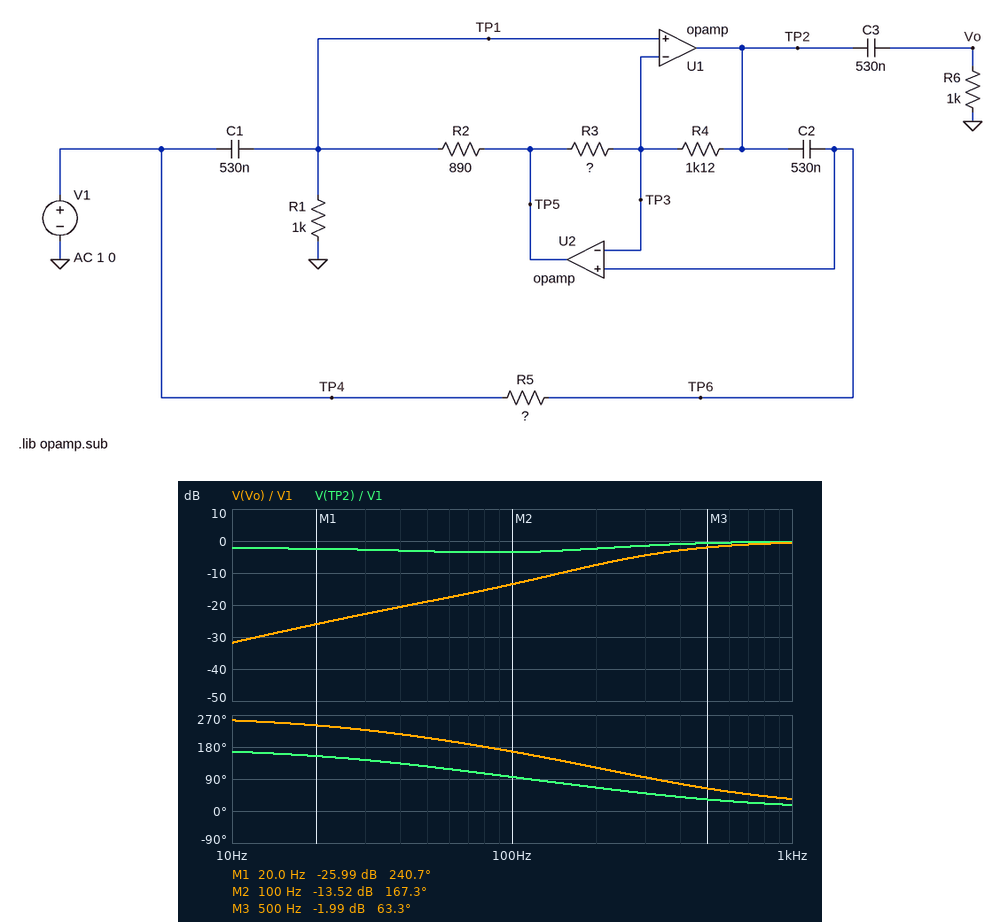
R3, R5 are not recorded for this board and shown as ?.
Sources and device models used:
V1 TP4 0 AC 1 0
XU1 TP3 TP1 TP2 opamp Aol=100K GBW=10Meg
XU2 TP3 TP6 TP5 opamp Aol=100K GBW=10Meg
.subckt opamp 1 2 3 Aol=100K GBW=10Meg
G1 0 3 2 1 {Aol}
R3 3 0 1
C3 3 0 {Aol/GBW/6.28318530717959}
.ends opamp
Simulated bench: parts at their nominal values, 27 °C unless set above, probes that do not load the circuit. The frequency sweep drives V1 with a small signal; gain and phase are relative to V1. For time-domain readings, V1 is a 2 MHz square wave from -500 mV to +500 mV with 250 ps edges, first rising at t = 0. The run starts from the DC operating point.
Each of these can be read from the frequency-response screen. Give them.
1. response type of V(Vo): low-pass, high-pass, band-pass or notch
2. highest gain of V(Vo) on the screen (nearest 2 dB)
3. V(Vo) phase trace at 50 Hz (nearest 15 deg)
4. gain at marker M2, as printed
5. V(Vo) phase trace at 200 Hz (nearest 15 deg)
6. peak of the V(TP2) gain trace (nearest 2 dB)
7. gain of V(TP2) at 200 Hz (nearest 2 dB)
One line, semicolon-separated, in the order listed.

high-pass; 0 dB; 210 deg; -13.52 dB; 120 deg; 0 dB; -2 dB
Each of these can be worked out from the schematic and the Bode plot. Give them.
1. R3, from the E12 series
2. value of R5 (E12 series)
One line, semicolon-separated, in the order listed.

560 Ω; 3.9 kΩ
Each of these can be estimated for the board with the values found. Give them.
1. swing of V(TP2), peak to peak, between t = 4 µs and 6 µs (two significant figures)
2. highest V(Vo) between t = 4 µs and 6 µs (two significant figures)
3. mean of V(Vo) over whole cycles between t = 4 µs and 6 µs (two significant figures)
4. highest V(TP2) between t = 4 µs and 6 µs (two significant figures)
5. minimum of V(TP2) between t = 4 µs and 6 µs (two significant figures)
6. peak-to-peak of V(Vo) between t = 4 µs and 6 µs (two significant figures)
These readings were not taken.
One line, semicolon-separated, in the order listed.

1.5 V; 1.2 V; 490 mV; 1.6 V; 140 mV; 1.5 V
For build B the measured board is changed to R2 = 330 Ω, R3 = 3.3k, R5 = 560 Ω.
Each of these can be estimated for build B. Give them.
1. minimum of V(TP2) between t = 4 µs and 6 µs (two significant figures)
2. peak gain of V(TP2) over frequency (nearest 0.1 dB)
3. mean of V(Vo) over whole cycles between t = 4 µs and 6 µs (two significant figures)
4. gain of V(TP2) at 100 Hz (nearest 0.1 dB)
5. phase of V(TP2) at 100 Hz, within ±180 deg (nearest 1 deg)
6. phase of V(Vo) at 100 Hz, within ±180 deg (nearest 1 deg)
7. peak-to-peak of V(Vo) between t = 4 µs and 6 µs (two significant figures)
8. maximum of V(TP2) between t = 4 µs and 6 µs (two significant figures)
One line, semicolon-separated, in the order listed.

-590 mV; 0.4 dB; 490 mV; -1.0 dB; -1 deg; 70 deg; 1.3 V; 690 mV
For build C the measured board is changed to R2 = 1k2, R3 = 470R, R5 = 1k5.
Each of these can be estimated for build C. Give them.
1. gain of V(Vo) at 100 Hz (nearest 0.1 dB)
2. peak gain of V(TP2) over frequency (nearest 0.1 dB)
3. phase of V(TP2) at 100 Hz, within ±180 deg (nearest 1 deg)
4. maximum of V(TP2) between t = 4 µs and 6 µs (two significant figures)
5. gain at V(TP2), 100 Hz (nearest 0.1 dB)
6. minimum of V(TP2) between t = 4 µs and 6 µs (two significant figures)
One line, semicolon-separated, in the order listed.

-6.3 dB; 5.4 dB; 110 deg; 2.2 V; 3.7 dB; 670 mV
